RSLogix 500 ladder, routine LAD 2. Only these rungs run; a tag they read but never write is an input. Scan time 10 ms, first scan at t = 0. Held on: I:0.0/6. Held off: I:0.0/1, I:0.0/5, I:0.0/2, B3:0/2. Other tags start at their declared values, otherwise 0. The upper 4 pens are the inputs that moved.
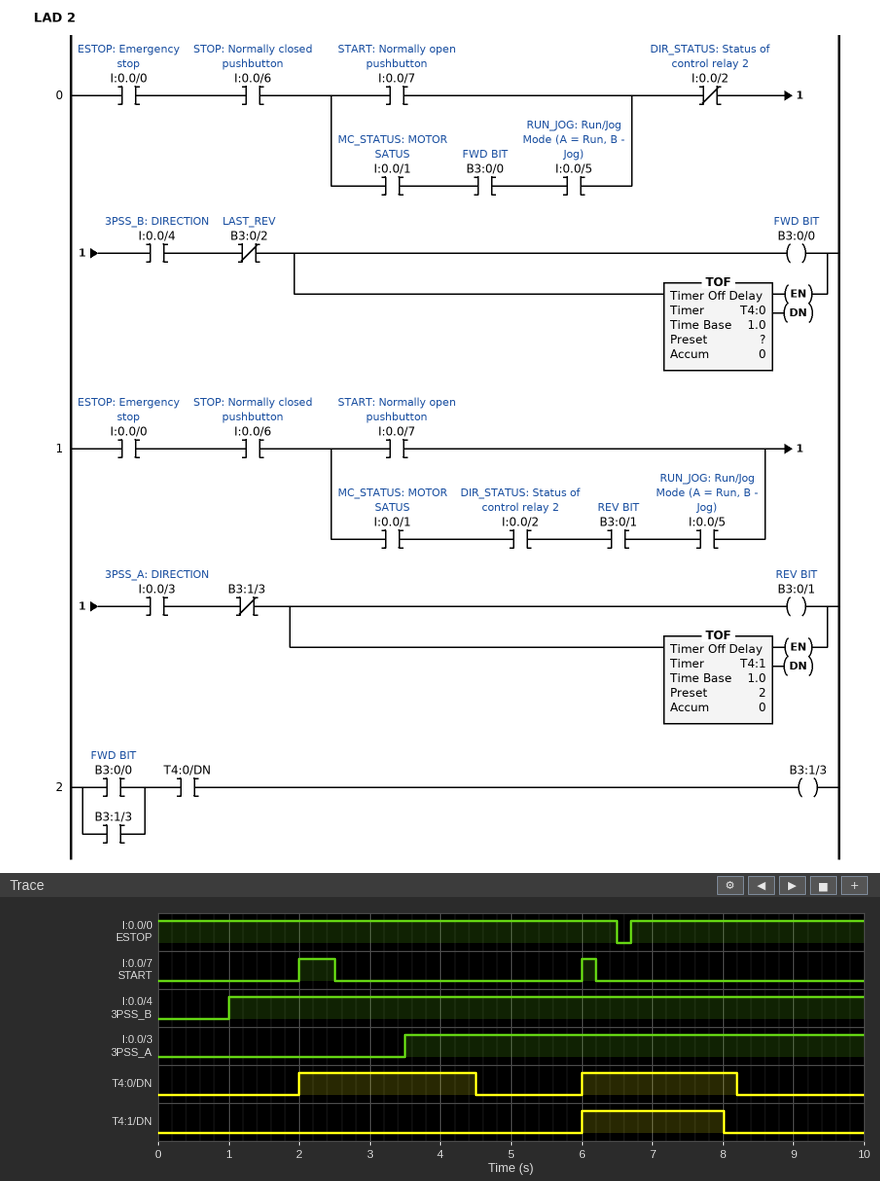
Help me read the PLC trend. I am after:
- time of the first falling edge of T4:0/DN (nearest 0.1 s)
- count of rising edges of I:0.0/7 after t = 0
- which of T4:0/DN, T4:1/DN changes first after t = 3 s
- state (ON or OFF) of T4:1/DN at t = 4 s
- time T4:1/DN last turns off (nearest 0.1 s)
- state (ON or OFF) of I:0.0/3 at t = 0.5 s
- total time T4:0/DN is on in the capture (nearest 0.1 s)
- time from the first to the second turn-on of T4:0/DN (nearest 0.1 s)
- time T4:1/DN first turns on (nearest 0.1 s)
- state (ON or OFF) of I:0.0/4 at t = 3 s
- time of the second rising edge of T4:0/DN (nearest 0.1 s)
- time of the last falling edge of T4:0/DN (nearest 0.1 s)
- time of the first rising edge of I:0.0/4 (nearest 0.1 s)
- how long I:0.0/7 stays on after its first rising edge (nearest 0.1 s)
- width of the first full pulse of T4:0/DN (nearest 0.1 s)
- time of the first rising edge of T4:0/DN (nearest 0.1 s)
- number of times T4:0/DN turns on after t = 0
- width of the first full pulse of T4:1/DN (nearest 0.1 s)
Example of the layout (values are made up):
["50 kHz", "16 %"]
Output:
["4.5 s", "2", "T4:0/DN", "OFF", "8.0 s", "OFF", "4.7 s", "4.0 s", "6.0 s", "ON", "6.0 s", "8.2 s", "1.0 s", "0.5 s", "2.5 s", "2.0 s", "2", "2.0 s"]
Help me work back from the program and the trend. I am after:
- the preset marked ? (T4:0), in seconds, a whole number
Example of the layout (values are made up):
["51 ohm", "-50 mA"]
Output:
["2 s"]
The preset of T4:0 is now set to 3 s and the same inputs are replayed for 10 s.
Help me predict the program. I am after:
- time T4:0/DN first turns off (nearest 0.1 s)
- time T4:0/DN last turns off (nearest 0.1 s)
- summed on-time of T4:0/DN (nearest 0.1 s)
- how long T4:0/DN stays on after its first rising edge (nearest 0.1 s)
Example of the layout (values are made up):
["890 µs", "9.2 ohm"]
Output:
["5.5 s", "9.2 s", "6.7 s", "3.5 s"]
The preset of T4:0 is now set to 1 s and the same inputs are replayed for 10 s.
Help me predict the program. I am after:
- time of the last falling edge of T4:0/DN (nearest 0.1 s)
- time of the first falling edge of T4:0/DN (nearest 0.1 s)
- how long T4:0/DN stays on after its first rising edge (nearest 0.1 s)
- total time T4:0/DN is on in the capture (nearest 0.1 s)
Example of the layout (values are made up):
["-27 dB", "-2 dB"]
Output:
["7.2 s", "3.5 s", "1.5 s", "2.7 s"]
